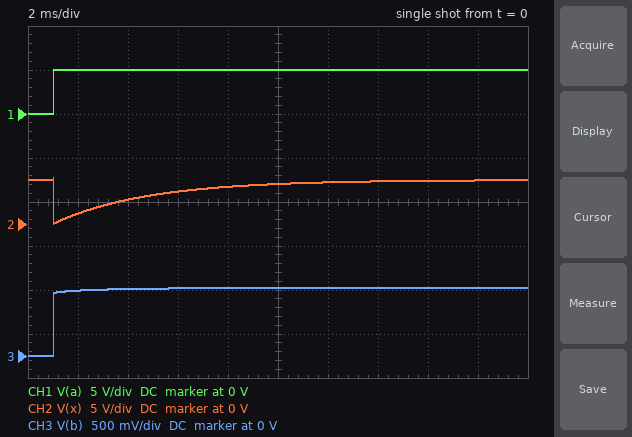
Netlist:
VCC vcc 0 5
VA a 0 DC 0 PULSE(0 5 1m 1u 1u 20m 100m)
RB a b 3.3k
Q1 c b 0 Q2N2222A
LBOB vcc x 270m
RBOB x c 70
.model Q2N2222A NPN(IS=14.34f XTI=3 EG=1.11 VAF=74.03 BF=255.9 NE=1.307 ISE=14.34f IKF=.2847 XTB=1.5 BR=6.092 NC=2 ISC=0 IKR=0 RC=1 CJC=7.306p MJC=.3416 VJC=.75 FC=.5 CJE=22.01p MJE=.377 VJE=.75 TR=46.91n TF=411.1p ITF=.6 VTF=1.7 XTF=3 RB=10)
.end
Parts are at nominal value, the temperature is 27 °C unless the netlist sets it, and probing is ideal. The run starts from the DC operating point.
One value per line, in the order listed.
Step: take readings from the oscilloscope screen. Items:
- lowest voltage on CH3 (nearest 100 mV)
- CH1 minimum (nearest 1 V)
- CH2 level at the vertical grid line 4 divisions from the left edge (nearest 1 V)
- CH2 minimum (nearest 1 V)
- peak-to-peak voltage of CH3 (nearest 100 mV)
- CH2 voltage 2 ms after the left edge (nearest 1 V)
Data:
0 V
0 V
4 V
0 V
800 mV
1 V
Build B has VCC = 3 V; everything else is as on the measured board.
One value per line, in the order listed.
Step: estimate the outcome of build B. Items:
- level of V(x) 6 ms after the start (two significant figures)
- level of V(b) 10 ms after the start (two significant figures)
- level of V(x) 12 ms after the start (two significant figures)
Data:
2.2 V
760 mV
2.8 V
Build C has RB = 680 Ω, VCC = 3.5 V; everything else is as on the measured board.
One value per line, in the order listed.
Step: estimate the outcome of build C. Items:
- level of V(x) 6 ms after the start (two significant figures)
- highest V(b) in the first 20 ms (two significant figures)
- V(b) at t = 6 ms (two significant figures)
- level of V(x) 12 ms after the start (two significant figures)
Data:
2.6 V
830 mV
820 mV
3.3 V
